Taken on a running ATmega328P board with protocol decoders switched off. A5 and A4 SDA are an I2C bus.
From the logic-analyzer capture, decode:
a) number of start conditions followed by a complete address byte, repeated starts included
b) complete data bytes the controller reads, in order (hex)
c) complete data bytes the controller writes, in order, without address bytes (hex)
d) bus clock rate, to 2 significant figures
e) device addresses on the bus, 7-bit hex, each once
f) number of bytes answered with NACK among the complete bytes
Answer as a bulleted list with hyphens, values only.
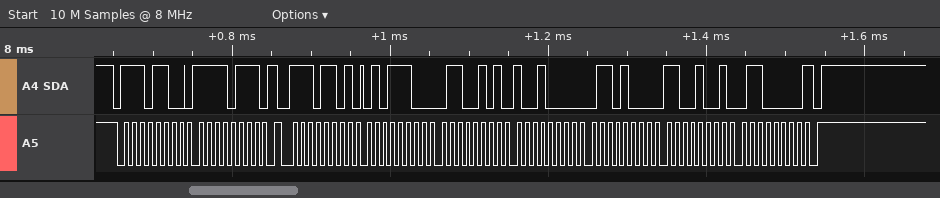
- 2
- 5C 65 90 68 C9 60
- F7
- 100 kHz
- 0x76
- 1
